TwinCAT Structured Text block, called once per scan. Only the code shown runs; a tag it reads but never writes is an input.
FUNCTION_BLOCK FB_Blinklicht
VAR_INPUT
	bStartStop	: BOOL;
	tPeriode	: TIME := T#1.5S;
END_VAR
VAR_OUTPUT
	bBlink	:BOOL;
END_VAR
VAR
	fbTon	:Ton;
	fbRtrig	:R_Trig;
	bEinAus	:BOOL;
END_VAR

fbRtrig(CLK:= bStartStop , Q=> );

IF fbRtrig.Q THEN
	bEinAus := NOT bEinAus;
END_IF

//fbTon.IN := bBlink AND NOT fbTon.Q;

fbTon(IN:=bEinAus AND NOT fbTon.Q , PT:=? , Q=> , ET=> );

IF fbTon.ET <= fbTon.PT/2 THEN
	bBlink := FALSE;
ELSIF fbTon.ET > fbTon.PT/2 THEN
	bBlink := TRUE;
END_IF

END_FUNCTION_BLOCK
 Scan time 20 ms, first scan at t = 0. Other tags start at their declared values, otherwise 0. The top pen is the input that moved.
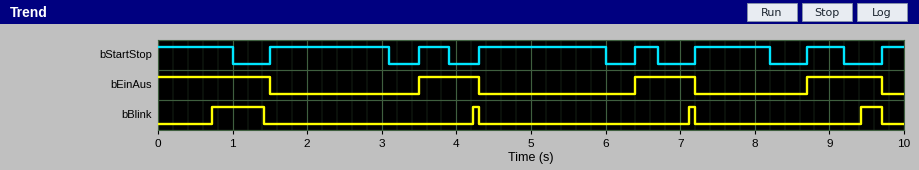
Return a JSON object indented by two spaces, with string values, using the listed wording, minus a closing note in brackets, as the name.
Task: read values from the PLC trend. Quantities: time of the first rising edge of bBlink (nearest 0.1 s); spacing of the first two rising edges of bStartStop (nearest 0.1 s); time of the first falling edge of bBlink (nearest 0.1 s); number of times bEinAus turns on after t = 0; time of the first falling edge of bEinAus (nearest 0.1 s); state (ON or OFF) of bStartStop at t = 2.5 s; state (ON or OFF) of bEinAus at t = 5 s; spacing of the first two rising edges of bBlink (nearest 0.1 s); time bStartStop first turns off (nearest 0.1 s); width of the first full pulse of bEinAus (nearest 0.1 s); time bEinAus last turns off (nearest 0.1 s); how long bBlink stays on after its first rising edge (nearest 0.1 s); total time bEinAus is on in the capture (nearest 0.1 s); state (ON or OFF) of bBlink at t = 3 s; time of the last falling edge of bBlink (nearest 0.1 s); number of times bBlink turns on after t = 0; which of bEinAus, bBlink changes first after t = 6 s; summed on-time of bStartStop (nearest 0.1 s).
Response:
{
  "time of the first rising edge of bBlink": "0.7 s",
  "spacing of the first two rising edges of bStartStop": "2.0 s",
  "time of the first falling edge of bBlink": "1.4 s",
  "number of times bEinAus turns on after t = 0": "3",
  "time of the first falling edge of bEinAus": "1.5 s",
  "state (ON or OFF) of bStartStop at t = 2.5 s": "ON",
  "state (ON or OFF) of bEinAus at t = 5 s": "OFF",
  "spacing of the first two rising edges of bBlink": "3.5 s",
  "time bStartStop first turns off": "1.0 s",
  "width of the first full pulse of bEinAus": "0.8 s",
  "time bEinAus last turns off": "9.7 s",
  "how long bBlink stays on after its first rising edge": "0.7 s",
  "total time bEinAus is on in the capture": "4.1 s",
  "state (ON or OFF) of bBlink at t = 3 s": "OFF",
  "time of the last falling edge of bBlink": "9.7 s",
  "number of times bBlink turns on after t = 0": "4",
  "which of bEinAus, bBlink changes first after t = 6 s": "bEinAus",
  "summed on-time of bStartStop": "6.8 s"
}
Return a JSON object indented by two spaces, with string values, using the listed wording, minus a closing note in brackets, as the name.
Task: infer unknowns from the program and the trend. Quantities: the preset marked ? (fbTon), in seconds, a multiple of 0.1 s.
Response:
{
  "the preset marked ? (fbTon), in seconds, a multiple of 0.1 s": "1.4 s"
}
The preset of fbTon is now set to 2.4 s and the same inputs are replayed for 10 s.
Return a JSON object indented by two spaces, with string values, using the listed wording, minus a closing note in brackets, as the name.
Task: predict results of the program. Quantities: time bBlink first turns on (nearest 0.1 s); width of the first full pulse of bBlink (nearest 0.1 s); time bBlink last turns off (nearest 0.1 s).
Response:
{
  "time bBlink first turns on": "1.2 s",
  "width of the first full pulse of bBlink": "0.3 s",
  "time bBlink last turns off": "1.5 s"
}
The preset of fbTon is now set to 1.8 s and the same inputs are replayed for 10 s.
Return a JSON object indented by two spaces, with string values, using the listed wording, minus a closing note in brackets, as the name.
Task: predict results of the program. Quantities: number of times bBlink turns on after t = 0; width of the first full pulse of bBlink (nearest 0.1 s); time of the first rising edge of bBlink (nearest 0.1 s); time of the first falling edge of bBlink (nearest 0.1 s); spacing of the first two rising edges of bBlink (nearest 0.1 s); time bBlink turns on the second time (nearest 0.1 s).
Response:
{
  "number of times bBlink turns on after t = 0": "2",
  "width of the first full pulse of bBlink": "0.6 s",
  "time of the first rising edge of bBlink": "0.9 s",
  "time of the first falling edge of bBlink": "1.5 s",
  "spacing of the first two rising edges of bBlink": "8.7 s",
  "time bBlink turns on the second time": "9.6 s"
}
